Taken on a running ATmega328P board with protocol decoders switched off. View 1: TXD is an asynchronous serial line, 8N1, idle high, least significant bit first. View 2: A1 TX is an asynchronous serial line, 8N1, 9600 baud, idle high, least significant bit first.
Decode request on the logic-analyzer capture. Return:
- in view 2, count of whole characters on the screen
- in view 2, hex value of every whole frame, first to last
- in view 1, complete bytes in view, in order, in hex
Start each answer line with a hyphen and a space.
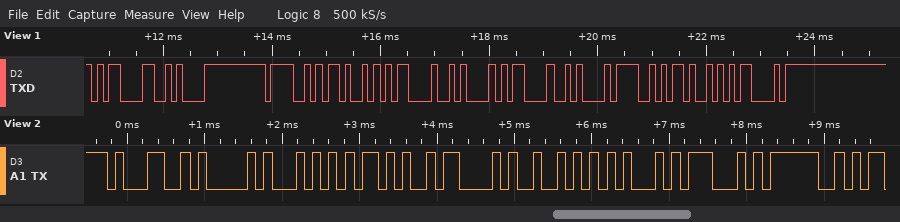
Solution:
- 9
- 0x31 0x41 0x54 0x2B 0x43 0x52 0x45 0x47 0x3F
- 0D 0A 4F 4B 0D 0A 0D 0A 4F 4B 0D FF
